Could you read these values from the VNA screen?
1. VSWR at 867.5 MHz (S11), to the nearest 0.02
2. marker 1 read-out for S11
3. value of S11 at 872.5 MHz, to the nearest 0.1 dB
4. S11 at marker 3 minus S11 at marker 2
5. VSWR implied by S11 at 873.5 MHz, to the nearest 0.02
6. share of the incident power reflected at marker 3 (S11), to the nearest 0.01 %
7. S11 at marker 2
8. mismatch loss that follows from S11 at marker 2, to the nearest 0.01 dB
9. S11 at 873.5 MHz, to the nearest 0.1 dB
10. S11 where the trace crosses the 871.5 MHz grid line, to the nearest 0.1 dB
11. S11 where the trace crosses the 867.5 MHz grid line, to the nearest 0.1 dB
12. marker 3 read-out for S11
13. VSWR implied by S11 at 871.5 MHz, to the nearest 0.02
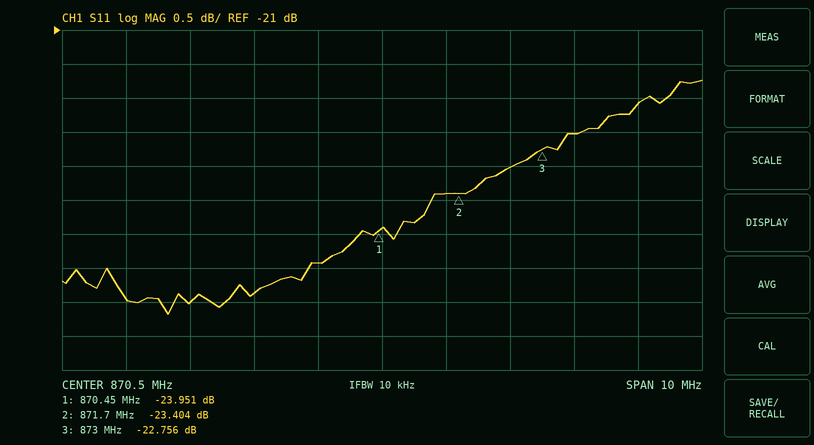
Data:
1.12
-23.951 dB
-23.0 dB
0.648 dB
1.16
0.53 %
-23.404 dB
0.02 dB
-22.5 dB
-23.4 dB
-25.0 dB
-22.756 dB
1.14
